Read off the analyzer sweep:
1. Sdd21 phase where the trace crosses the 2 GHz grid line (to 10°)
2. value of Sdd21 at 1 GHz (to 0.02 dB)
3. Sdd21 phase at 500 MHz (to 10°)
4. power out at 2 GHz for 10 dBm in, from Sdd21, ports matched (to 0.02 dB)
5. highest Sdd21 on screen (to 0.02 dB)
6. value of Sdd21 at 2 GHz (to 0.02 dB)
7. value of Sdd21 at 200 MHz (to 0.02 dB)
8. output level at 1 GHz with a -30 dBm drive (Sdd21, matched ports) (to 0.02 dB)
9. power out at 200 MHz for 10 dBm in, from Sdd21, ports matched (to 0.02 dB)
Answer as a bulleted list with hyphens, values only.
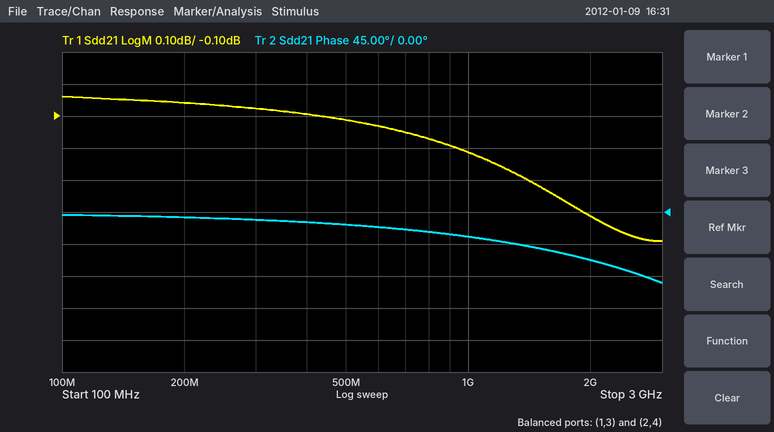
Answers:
- -70°
- -0.22 dB
- -20°
- 9.58 dBm
- -0.04 dB
- -0.42 dB
- -0.06 dB
- -30.22 dBm
- 9.94 dBm
